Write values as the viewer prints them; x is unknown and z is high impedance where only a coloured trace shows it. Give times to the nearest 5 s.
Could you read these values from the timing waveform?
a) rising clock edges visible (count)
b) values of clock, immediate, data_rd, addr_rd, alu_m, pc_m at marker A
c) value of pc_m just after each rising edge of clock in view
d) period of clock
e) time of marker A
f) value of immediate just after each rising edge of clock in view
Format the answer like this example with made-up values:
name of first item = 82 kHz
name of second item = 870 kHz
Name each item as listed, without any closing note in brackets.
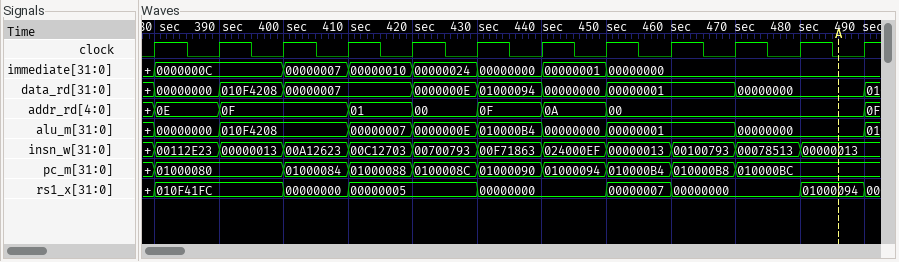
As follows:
rising clock edges visible = 12
values of clock, immediate, data_rd, addr_rd, alu_m, pc_m at marker A = clock=0, immediate=00000000, data_rd=00000000, addr_rd=00, alu_m=00000000, pc_m=010000BC
value of pc_m just after each rising edge of clock in view = 01000080, 01000080, 01000084, 01000088, 0100008C, 01000090, 01000094, 010000B4, 010000B8, 010000BC, 010000BC, 010000BC
period of clock = 10 s
time of marker A = 485 s
value of immediate just after each rising edge of clock in view = 0000000C, 0000000C, 00000007, 00000010, 00000024, 00000000, 00000001, 00000000, 00000000, 00000000, 00000000, 00000000
